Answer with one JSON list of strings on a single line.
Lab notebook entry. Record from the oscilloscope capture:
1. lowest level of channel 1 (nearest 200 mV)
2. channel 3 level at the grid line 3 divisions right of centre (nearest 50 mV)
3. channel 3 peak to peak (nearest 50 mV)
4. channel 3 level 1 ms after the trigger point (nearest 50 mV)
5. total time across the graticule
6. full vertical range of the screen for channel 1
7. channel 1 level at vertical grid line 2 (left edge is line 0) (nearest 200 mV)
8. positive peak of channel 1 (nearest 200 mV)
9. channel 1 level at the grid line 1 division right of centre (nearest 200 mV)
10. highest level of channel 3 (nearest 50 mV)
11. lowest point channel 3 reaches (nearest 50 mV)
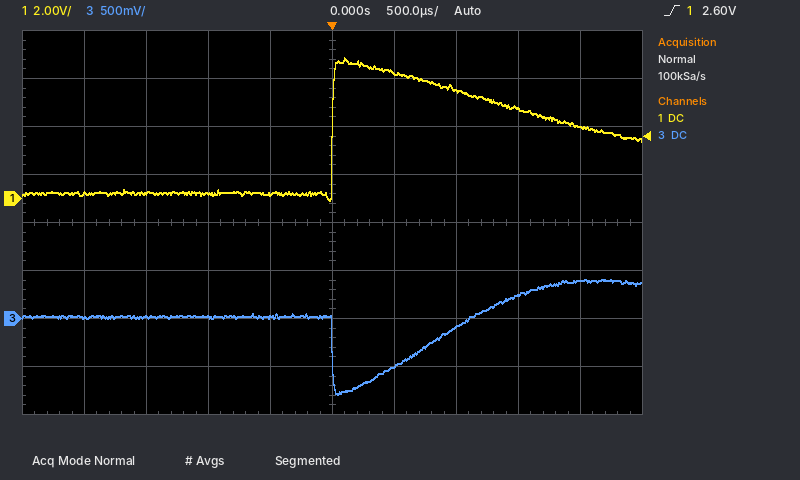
["0.0 V", "250 mV", "1.20 V", "-100 mV", "5 ms", "16 V", "200 mV", "5.8 V", "5.2 V", "400 mV", "-800 mV"]
